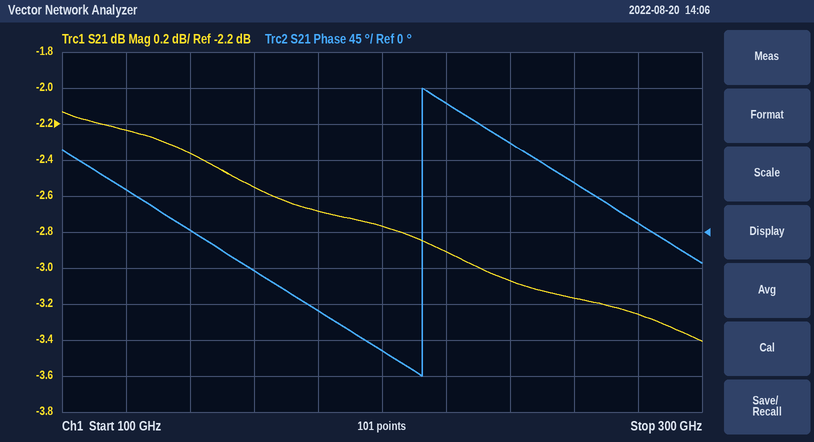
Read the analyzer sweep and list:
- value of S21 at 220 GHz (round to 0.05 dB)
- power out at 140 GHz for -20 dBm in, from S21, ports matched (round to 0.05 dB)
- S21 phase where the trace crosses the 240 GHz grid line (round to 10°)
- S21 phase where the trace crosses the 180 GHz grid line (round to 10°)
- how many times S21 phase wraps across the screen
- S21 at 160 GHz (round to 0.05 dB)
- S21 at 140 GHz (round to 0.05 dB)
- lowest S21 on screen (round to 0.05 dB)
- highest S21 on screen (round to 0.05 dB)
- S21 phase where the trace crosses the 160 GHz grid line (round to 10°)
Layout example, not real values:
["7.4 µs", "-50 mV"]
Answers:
["-2.90 dB", "-22.35 dBm", "110°", "-100°", "1", "-2.55 dB", "-2.35 dB", "-3.40 dB", "-2.15 dB", "-50°"]
